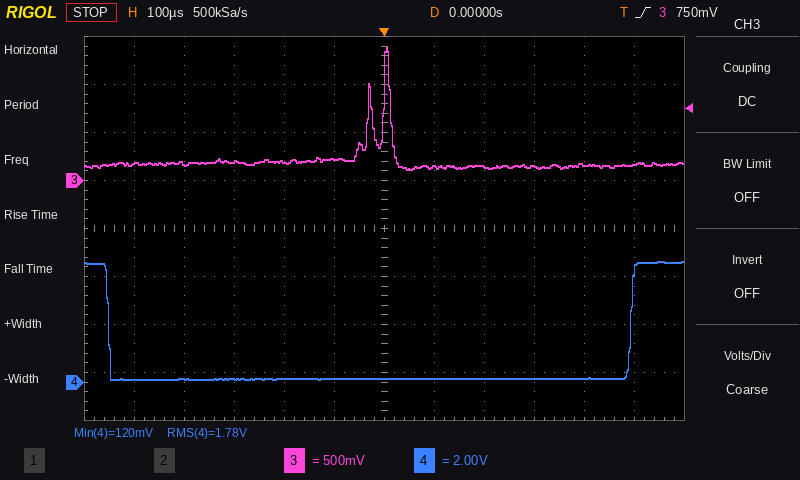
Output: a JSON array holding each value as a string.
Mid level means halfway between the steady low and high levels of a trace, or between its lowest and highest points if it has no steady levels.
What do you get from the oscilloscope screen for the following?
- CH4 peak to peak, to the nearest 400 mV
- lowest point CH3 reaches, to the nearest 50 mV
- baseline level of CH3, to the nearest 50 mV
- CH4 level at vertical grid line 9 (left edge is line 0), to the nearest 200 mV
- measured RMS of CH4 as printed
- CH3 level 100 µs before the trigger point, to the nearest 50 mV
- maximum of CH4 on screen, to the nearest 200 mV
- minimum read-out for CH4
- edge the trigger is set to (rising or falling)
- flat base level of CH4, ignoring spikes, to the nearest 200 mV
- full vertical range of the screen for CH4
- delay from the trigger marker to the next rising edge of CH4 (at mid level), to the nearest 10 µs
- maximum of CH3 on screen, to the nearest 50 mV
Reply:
["4.8 V", "100 mV", "150 mV", "200 mV", "1.78 V", "200 mV", "5.0 V", "120 mV", "rising", "200 mV", "16 V", "490 µs", "1.40 V"]
